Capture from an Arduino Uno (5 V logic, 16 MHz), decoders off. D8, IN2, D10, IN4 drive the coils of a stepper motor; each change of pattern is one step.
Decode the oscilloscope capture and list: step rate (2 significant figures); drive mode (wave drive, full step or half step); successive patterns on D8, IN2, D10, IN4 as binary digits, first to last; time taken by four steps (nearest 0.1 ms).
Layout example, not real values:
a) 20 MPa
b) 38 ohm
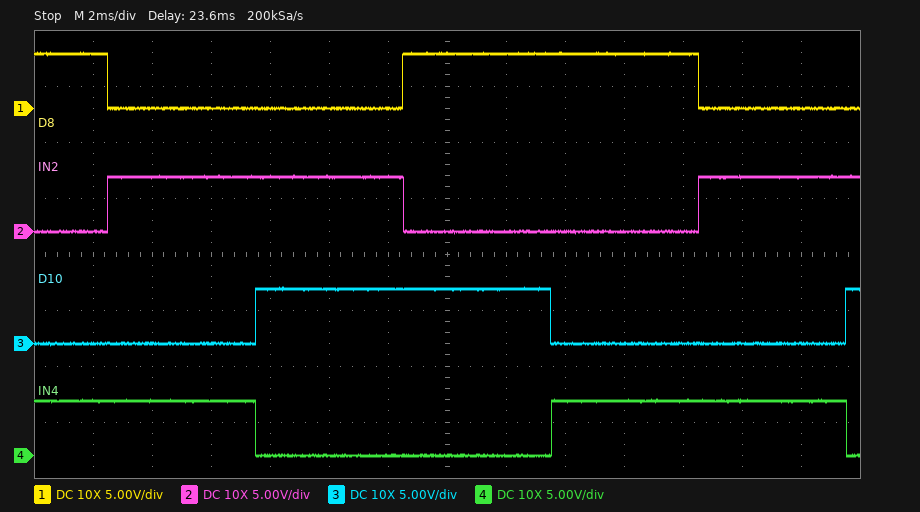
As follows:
a) 200 steps/s
b) full step
c) 1001 0101 0110 1010 1001 0101 0110
d) 20.0 ms
